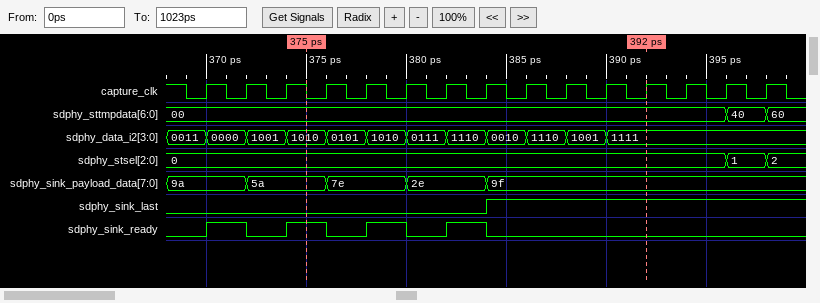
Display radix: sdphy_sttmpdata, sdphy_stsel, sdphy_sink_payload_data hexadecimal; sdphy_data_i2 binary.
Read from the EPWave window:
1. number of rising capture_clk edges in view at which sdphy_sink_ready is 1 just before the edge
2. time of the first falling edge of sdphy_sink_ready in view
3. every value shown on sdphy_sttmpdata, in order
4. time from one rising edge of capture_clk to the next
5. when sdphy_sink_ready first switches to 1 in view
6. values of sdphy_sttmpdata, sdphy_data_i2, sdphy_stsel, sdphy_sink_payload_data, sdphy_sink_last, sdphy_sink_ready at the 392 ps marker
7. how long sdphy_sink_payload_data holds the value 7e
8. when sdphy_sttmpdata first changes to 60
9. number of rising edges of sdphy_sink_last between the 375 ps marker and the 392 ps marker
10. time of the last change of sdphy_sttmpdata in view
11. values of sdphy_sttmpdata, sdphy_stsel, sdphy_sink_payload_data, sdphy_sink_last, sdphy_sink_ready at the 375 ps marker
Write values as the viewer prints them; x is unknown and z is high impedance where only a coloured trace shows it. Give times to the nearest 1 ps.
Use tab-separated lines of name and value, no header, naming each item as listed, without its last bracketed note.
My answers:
number of rising capture_clk edges in view at which sdphy_sink_ready is 1 just before the edge	4
time of the first falling edge of sdphy_sink_ready in view	372 ps
every value shown on sdphy_sttmpdata, in order	00, 40, 60
time from one rising edge of capture_clk to the next	2 ps
when sdphy_sink_ready first switches to 1 in view	370 ps
values of sdphy_sttmpdata, sdphy_data_i2, sdphy_stsel, sdphy_sink_payload_data, sdphy_sink_last, sdphy_sink_ready at the 392 ps marker	sdphy_sttmpdata=00, sdphy_data_i2=1111, sdphy_stsel=0, sdphy_sink_payload_data=9f, sdphy_sink_last=1, sdphy_sink_ready=0
how long sdphy_sink_payload_data holds the value 7e	4 ps
when sdphy_sttmpdata first changes to 60	398 ps
number of rising edges of sdphy_sink_last between the 375 ps marker and the 392 ps marker	1
time of the last change of sdphy_sttmpdata in view	398 ps
values of sdphy_sttmpdata, sdphy_stsel, sdphy_sink_payload_data, sdphy_sink_last, sdphy_sink_ready at the 375 ps marker	sdphy_sttmpdata=00, sdphy_stsel=0, sdphy_sink_payload_data=5a, sdphy_sink_last=0, sdphy_sink_ready=1
